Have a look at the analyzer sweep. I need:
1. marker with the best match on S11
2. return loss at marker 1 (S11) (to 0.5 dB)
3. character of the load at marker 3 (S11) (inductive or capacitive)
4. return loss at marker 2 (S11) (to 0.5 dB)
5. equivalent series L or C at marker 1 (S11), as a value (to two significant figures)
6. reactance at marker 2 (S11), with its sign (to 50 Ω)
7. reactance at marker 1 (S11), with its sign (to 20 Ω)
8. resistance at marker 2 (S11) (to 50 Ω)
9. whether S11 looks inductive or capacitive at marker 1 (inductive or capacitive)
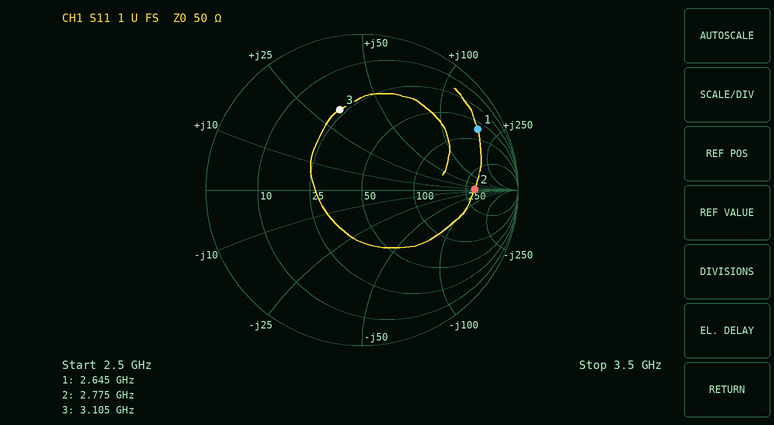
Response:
marker 3
1.5 dB
inductive
3.0 dB
11 nH
0 Ω
+180 Ω
300 Ω
inductive
